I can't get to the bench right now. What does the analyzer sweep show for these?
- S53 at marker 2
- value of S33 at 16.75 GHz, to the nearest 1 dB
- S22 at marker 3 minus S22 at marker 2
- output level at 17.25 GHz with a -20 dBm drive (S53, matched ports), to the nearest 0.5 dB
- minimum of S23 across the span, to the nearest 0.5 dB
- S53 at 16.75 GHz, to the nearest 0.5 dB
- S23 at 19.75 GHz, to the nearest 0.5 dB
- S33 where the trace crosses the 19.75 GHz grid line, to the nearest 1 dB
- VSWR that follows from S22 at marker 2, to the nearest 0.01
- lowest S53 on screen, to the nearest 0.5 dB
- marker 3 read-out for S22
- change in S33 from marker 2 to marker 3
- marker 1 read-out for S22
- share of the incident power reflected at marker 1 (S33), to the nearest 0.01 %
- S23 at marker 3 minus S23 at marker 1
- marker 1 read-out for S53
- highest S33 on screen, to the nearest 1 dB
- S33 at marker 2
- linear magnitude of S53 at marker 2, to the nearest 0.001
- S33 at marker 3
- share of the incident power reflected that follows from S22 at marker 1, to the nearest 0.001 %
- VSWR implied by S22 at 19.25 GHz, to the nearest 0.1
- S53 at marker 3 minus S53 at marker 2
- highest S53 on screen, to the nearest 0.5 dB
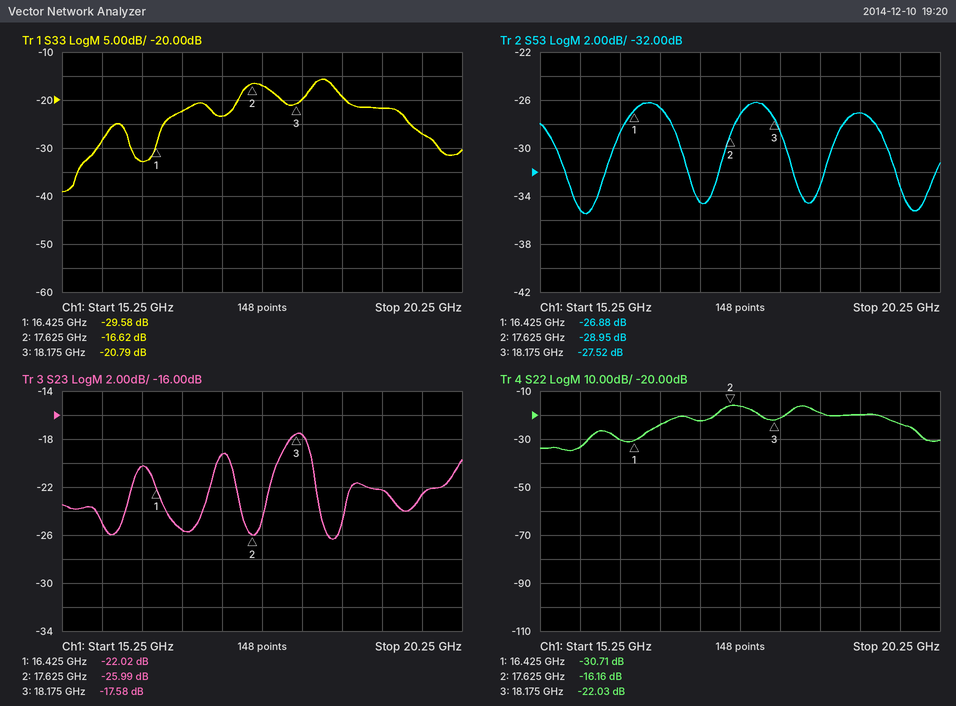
-28.95 dB
-22 dB
-5.87 dB
-54.5 dBm
-26.5 dB
-26.5 dB
-22.5 dB
-27 dB
1.37
-35.5 dB
-22.03 dB
-4.17 dB
-30.71 dB
0.11 %
4.44 dB
-26.88 dB
-16 dB
-16.62 dB
0.036
-20.79 dB
0.085 %
1.2
1.43 dB
-26.0 dB
